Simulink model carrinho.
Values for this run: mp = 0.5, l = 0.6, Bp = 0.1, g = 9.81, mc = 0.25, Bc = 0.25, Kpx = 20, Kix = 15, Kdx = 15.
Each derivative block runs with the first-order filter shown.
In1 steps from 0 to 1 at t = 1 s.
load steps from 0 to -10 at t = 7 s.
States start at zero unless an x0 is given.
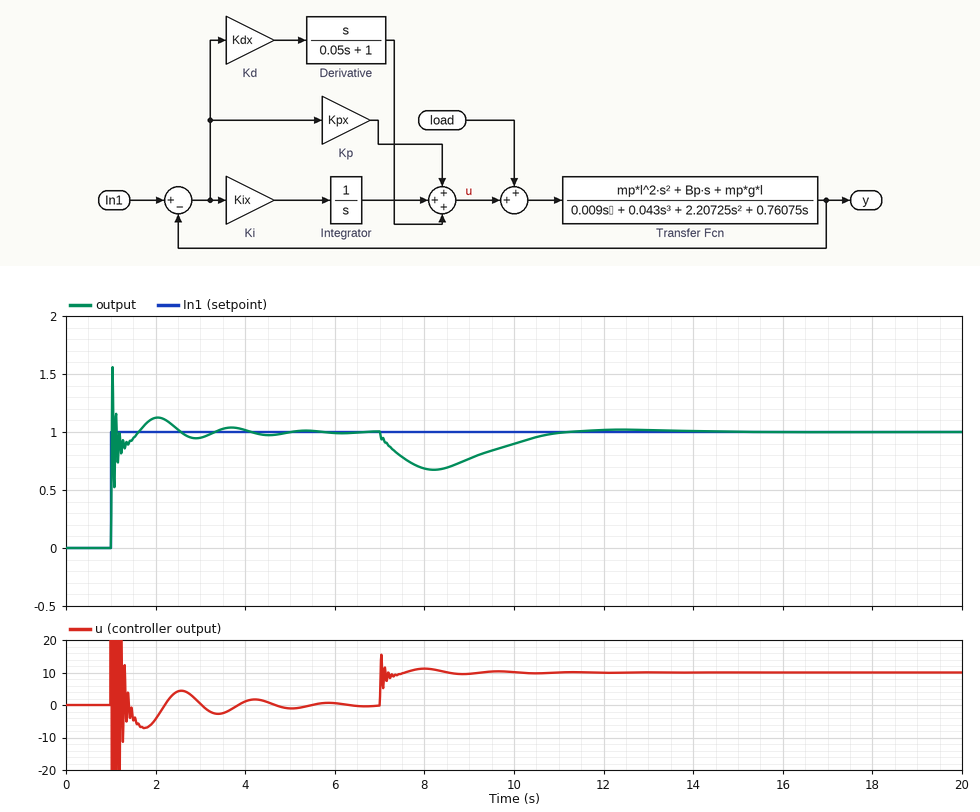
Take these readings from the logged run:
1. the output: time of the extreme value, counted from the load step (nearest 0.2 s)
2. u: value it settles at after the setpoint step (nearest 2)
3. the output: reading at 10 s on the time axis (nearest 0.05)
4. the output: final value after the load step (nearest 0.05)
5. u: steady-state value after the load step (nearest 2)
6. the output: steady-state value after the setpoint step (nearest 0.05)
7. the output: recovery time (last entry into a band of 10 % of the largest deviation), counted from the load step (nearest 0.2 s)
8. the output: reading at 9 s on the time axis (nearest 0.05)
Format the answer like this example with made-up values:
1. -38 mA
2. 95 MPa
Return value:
1. 1.2 s
2. 0
3. 0.90
4. 1.00
5. 10
6. 1.00
7. 3.6 s
8. 0.75
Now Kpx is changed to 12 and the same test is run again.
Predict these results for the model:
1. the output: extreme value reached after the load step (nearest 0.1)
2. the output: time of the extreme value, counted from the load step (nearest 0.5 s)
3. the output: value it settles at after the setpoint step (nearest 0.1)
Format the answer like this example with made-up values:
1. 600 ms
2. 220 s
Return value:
1. 0.6
2. 1.5 s
3. 1.0
